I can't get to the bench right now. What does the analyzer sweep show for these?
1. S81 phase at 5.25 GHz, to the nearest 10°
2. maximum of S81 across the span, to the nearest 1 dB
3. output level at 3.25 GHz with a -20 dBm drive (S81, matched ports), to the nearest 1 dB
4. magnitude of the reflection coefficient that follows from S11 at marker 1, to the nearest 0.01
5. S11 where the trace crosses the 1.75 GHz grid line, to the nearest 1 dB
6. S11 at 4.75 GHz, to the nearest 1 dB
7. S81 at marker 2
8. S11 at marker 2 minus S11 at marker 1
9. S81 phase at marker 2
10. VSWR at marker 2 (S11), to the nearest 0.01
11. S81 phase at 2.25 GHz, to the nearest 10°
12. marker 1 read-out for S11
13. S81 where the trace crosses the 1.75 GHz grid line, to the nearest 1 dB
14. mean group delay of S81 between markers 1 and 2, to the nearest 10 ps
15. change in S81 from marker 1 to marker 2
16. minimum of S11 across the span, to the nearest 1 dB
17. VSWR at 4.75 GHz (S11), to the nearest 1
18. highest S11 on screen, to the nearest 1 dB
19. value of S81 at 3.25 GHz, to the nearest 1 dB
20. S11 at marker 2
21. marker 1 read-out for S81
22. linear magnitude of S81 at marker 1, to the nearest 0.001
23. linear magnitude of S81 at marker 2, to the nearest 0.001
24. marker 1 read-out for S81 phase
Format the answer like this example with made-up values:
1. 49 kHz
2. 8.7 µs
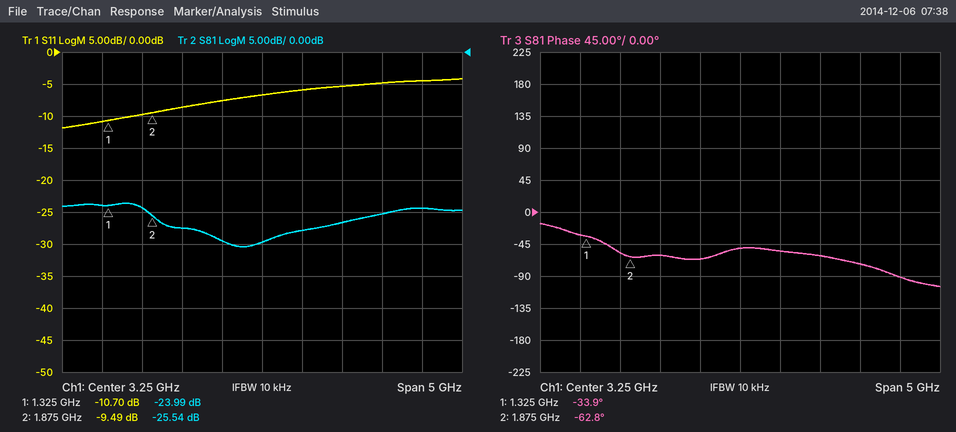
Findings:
1. -90°
2. -24 dB
3. -50 dBm
4. 0.29
5. -10 dB
6. -5 dB
7. -25.54 dB
8. 1.21 dB
9. -62.8°
10. 2.01
11. -60°
12. -10.70 dB
13. -24 dB
14. 150 ps
15. -1.55 dB
16. -12 dB
17. 4
18. -4 dB
19. -30 dB
20. -9.49 dB
21. -23.99 dB
22. 0.063
23. 0.053
24. -33.9°
